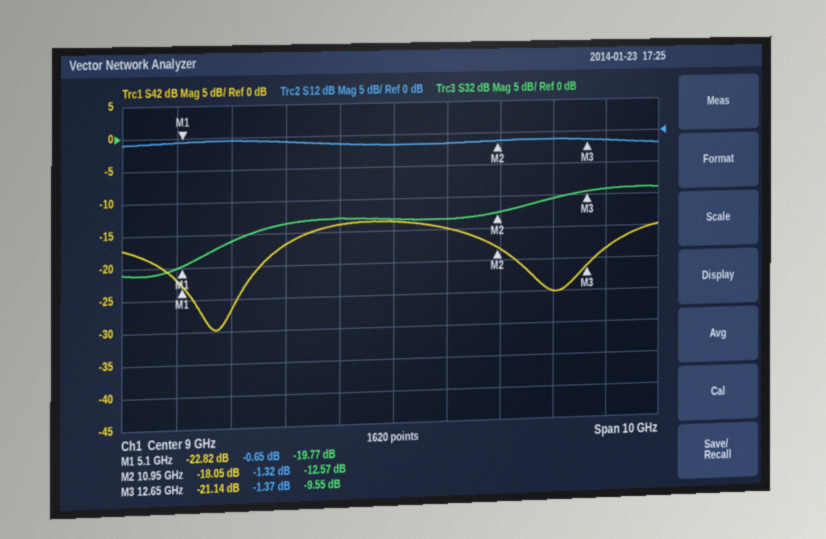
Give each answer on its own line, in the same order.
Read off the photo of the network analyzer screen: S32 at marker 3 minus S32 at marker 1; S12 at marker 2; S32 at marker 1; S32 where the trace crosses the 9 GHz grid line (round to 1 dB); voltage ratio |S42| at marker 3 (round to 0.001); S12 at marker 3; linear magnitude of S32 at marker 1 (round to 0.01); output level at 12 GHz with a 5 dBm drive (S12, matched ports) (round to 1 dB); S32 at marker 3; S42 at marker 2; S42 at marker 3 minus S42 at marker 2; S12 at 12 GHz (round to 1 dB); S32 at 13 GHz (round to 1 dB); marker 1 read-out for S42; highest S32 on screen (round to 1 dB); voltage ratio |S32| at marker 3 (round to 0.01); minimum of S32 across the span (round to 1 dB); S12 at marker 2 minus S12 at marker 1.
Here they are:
10.22 dB
-1.32 dB
-19.77 dB
-13 dB
0.088
-1.37 dB
0.10
4 dBm
-9.55 dB
-18.05 dB
-3.09 dB
-1 dB
-9 dB
-22.82 dB
-9 dB
0.33
-21 dB
-0.67 dB
